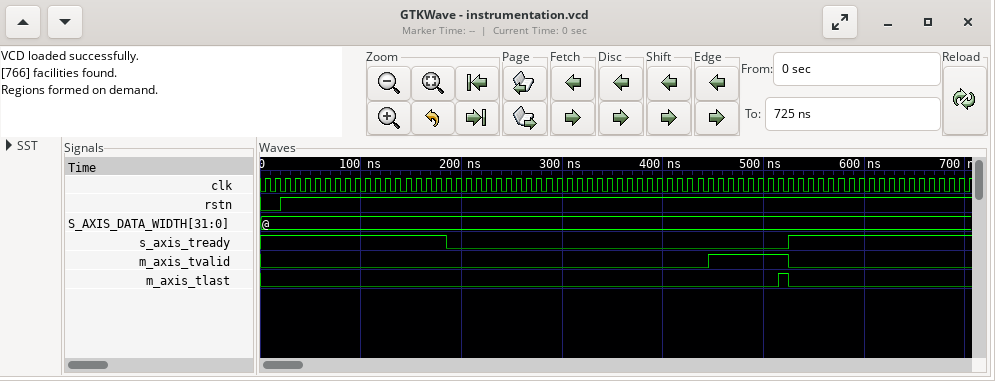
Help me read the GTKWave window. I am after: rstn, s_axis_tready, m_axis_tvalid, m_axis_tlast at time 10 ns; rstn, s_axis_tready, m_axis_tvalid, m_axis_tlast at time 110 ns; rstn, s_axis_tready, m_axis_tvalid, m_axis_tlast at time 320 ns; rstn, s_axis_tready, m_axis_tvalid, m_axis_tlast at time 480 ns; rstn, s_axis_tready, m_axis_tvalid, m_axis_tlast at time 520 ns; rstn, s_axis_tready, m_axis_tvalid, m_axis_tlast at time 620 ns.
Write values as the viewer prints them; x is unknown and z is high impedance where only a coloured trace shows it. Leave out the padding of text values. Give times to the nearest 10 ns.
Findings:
rstn=0, s_axis_tready=1, m_axis_tvalid=0, m_axis_tlast=0
rstn=1, s_axis_tready=1, m_axis_tvalid=0, m_axis_tlast=0
rstn=1, s_axis_tready=0, m_axis_tvalid=0, m_axis_tlast=0
rstn=1, s_axis_tready=0, m_axis_tvalid=1, m_axis_tlast=0
rstn=1, s_axis_tready=0, m_axis_tvalid=1, m_axis_tlast=1
rstn=1, s_axis_tready=1, m_axis_tvalid=0, m_axis_tlast=0
